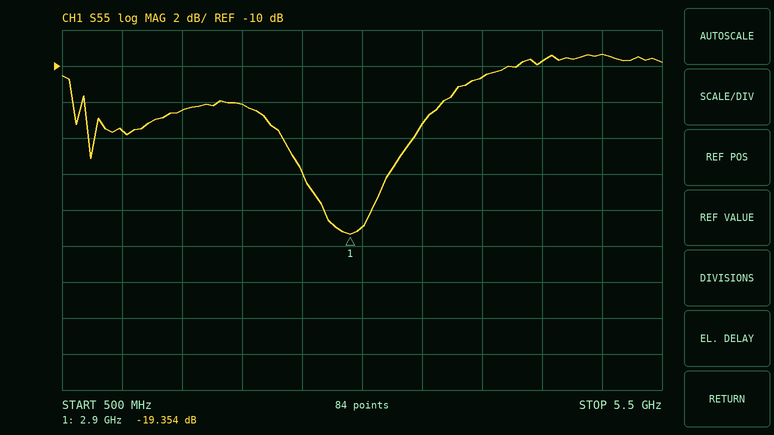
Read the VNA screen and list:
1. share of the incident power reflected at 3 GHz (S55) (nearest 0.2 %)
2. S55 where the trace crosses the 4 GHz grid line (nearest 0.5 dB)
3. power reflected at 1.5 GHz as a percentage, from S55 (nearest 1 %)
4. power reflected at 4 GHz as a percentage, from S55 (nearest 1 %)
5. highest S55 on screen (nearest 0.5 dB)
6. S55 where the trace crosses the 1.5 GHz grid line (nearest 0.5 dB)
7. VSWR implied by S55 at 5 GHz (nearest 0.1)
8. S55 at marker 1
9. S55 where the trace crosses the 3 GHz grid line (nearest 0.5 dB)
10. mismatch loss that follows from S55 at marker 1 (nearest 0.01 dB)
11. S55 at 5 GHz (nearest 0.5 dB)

1.2 %
-10.5 dB
6 %
9 %
-9.5 dB
-12.5 dB
2.0
-19.354 dB
-19.0 dB
0.05 dB
-9.5 dB
